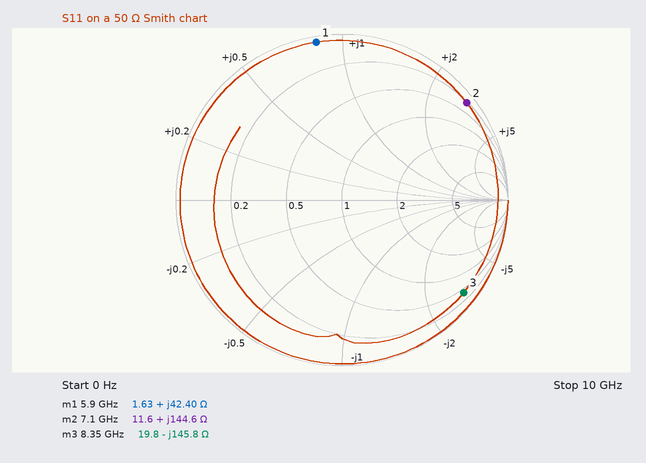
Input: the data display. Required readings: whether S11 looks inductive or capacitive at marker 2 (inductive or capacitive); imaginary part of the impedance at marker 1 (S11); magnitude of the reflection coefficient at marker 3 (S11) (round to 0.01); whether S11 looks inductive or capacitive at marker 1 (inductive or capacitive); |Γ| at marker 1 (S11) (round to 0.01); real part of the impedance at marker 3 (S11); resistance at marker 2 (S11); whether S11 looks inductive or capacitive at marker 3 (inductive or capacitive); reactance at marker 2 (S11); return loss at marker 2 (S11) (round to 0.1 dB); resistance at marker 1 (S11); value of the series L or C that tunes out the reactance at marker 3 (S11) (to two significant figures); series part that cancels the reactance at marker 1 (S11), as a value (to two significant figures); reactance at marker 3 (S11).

inductive
+42.40 Ω
0.92
inductive
0.96
19.8 Ω
11.6 Ω
capacitive
+144.6 Ω
0.4 dB
1.63 Ω
2.8 nH
640 fF
-145.8 Ω
